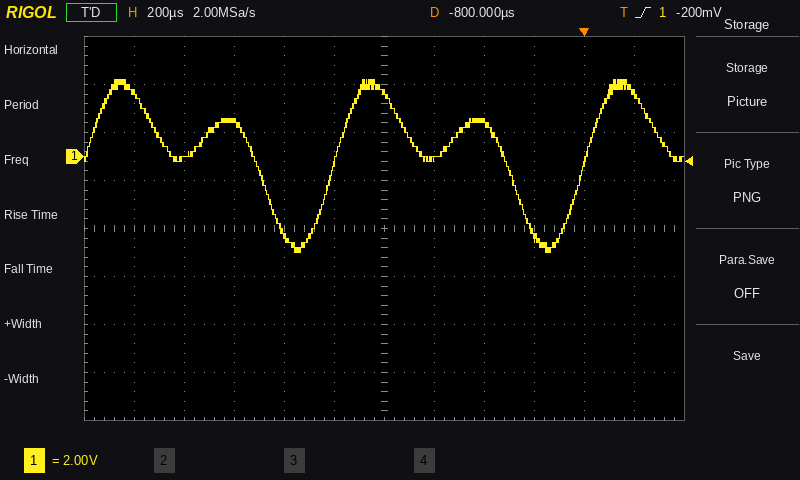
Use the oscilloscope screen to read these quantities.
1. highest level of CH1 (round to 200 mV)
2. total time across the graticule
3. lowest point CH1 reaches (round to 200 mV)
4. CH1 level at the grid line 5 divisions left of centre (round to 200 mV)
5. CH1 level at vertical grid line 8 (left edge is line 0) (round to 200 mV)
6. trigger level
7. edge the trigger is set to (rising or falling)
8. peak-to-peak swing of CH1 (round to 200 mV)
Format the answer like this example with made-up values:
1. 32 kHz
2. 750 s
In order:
1. 3.2 V
2. 2.4 ms
3. -4.0 V
4. 2.6 V
5. 1.4 V
6. -200 mV
7. rising
8. 7.2 V
